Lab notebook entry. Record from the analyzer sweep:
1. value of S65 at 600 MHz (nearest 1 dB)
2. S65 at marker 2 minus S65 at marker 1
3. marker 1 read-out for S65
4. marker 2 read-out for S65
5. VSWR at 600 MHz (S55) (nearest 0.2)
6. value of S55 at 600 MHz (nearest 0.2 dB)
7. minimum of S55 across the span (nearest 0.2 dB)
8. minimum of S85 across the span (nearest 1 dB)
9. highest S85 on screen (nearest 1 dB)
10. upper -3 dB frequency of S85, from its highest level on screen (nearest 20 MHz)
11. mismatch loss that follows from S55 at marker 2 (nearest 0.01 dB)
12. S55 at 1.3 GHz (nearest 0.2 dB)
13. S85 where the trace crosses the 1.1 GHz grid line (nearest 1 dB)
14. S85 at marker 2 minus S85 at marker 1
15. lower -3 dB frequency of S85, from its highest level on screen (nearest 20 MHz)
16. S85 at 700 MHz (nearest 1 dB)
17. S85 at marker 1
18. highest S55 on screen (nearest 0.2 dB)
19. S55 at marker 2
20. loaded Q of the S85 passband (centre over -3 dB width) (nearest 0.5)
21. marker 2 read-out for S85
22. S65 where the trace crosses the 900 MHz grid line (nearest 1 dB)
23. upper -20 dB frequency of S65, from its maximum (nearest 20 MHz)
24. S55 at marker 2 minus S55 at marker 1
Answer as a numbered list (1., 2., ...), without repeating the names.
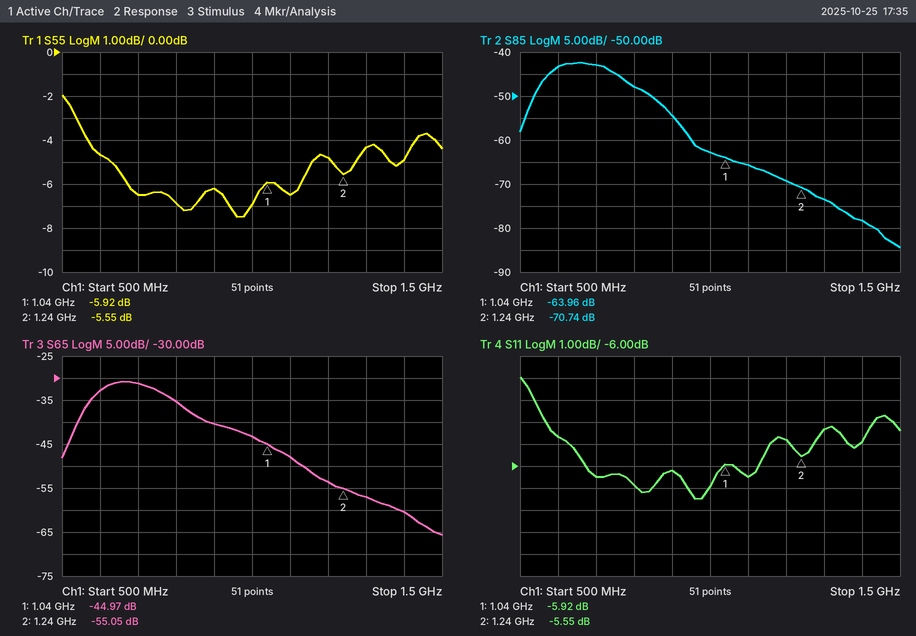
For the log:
1. -33 dB
2. -10.08 dB
3. -44.97 dB
4. -55.05 dB
5. 3.8
6. -4.6 dB
7. -7.4 dB
8. -84 dB
9. -42 dB
10. 760 MHz
11. 1.42 dB
12. -4.4 dB
13. -66 dB
14. -6.78 dB
15. 580 MHz
16. -43 dB
17. -63.96 dB
18. -2.0 dB
19. -5.55 dB
20. 3.5
21. -70.74 dB
22. -40 dB
23. 1.14 GHz
24. 0.37 dB
